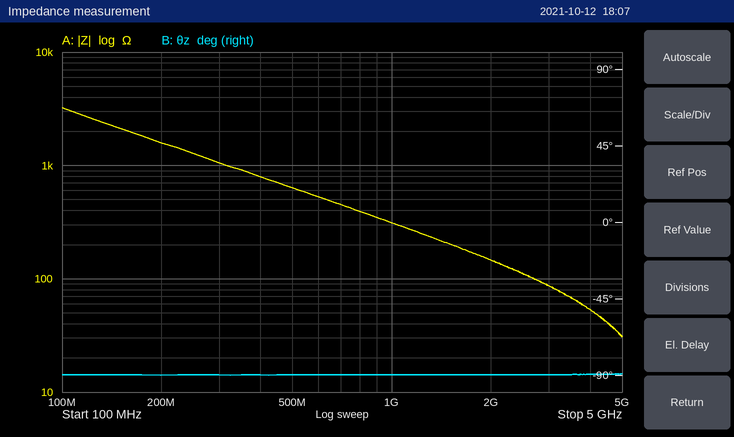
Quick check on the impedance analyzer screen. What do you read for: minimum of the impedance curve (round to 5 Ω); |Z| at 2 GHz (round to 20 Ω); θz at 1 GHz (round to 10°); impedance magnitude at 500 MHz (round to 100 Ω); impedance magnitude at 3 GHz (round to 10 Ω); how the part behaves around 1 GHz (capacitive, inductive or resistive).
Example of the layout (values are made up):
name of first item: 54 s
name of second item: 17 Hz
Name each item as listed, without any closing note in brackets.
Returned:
minimum of the impedance curve: 30 Ω
|Z| at 2 GHz: 140 Ω
θz at 1 GHz: -90°
impedance magnitude at 500 MHz: 600 Ω
impedance magnitude at 3 GHz: 90 Ω
how the part behaves around 1 GHz: capacitive
